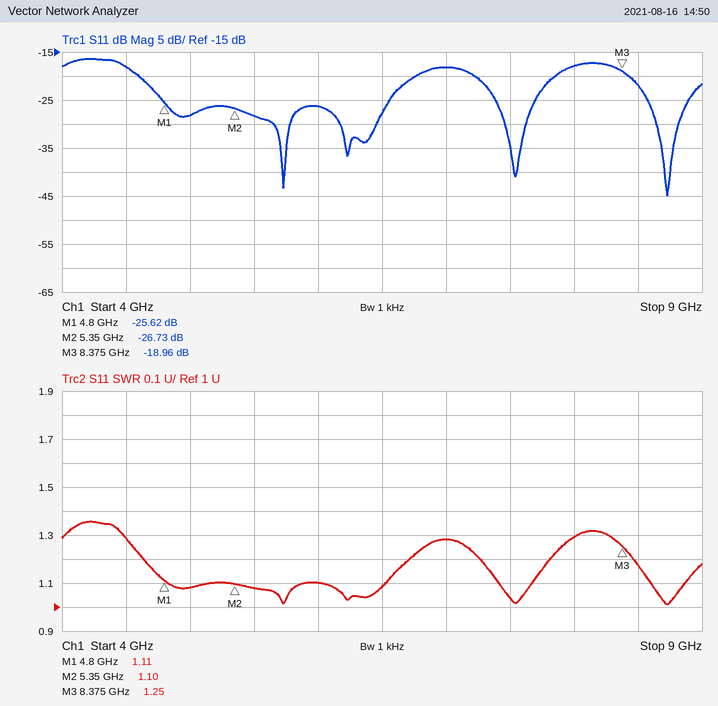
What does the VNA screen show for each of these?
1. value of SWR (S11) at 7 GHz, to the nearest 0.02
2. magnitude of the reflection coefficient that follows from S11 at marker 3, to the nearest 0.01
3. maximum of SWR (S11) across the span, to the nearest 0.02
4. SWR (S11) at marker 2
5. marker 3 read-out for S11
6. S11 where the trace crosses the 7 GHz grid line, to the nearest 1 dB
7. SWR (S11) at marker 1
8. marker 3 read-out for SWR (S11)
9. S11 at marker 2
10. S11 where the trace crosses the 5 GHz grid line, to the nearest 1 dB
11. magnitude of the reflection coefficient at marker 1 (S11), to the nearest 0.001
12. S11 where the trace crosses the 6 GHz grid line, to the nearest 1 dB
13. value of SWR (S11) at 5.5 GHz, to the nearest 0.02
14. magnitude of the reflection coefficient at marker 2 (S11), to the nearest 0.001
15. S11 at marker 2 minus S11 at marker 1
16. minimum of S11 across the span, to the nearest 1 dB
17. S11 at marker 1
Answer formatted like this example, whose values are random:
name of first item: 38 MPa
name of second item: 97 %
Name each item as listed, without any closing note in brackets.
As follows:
value of SWR (S11) at 7 GHz, to the nearest 0.02: 1.28
magnitude of the reflection coefficient that follows from S11 at marker 3, to the nearest 0.01: 0.11
maximum of SWR (S11) across the span, to the nearest 0.02: 1.36
SWR (S11) at marker 2: 1.10
marker 3 read-out for S11: -18.96 dB
S11 where the trace crosses the 7 GHz grid line, to the nearest 1 dB: -18 dB
SWR (S11) at marker 1: 1.11
marker 3 read-out for SWR: 1.25
S11 at marker 2: -26.73 dB
S11 where the trace crosses the 5 GHz grid line, to the nearest 1 dB: -28 dB
magnitude of the reflection coefficient at marker 1 (S11), to the nearest 0.001: 0.052
S11 where the trace crosses the 6 GHz grid line, to the nearest 1 dB: -26 dB
value of SWR (S11) at 5.5 GHz, to the nearest 0.02: 1.08
magnitude of the reflection coefficient at marker 2 (S11), to the nearest 0.001: 0.046
S11 at marker 2 minus S11 at marker 1: -1.11 dB
minimum of S11 across the span, to the nearest 1 dB: -45 dB
S11 at marker 1: -25.62 dB
